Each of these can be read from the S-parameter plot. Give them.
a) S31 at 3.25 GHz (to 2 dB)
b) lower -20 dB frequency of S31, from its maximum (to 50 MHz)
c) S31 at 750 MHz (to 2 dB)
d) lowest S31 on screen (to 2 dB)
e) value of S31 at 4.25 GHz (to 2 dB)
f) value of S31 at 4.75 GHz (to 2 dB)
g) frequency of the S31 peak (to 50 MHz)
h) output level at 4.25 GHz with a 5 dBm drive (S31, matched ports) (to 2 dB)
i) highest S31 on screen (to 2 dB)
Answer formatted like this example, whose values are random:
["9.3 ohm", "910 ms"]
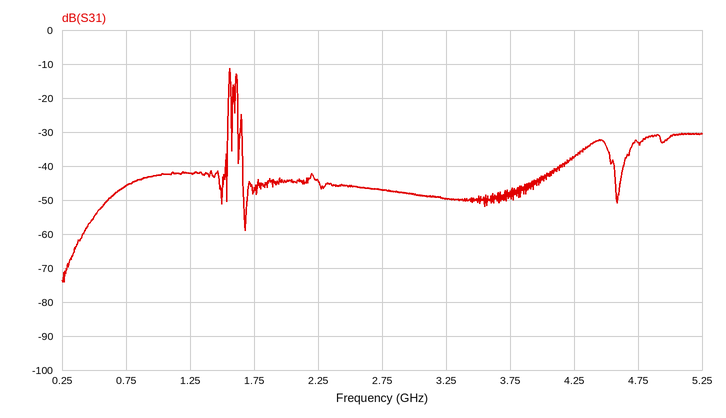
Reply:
["-50 dB", "1.55 GHz", "-46 dB", "-74 dB", "-38 dB", "-34 dB", "1.55 GHz", "-32 dBm", "-12 dB"]
